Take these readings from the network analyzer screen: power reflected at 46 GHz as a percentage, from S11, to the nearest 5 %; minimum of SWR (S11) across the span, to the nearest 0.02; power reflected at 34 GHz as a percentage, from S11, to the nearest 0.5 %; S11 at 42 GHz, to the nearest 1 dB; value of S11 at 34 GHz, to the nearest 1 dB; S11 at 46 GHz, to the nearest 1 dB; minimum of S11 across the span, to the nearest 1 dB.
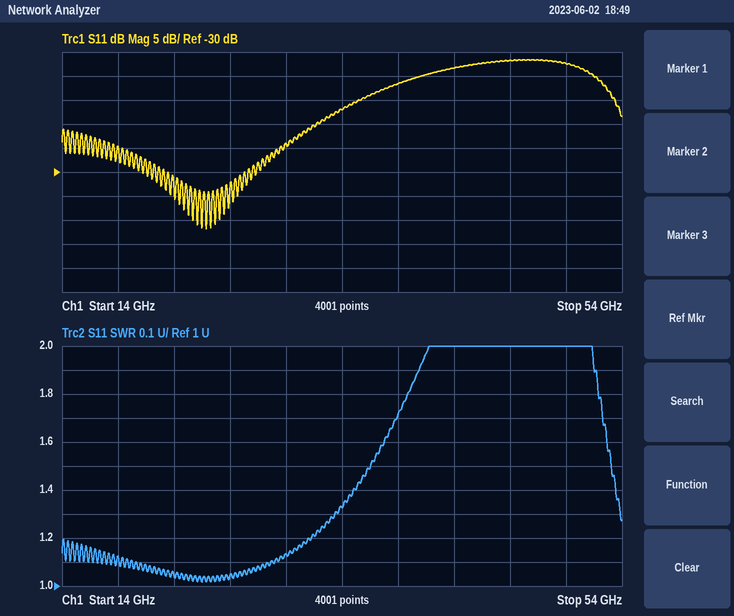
20 %
1.02
2.0 %
-8 dB
-17 dB
-7 dB
-42 dB
